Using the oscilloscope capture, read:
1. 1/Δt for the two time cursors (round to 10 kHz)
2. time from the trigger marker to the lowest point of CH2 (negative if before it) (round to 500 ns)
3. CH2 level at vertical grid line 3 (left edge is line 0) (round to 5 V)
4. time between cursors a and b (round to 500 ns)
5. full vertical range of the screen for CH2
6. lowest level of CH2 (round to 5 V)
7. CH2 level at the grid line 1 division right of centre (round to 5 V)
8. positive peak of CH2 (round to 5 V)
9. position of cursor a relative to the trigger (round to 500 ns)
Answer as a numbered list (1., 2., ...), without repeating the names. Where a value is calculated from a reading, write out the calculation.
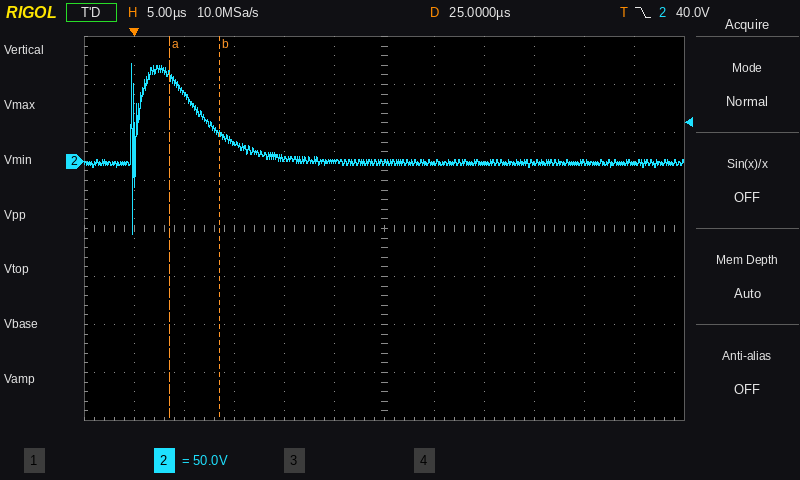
1. 1 / 5.0 µs ≈ 200 kHz
2. 0.0 µs
3. 20 V
4. 5.0 µs
5. 400 V
6. -75 V
7. 0 V
8. 100 V
9. +3.5 µs
